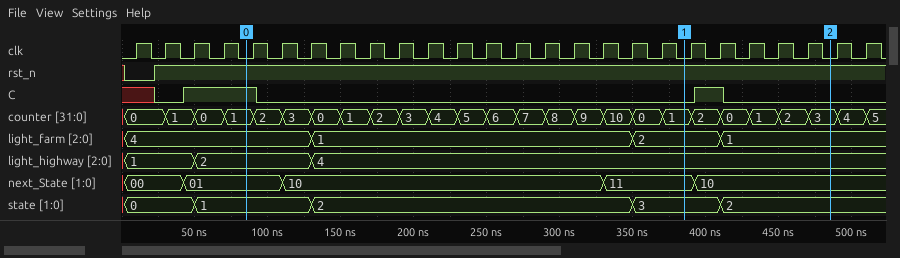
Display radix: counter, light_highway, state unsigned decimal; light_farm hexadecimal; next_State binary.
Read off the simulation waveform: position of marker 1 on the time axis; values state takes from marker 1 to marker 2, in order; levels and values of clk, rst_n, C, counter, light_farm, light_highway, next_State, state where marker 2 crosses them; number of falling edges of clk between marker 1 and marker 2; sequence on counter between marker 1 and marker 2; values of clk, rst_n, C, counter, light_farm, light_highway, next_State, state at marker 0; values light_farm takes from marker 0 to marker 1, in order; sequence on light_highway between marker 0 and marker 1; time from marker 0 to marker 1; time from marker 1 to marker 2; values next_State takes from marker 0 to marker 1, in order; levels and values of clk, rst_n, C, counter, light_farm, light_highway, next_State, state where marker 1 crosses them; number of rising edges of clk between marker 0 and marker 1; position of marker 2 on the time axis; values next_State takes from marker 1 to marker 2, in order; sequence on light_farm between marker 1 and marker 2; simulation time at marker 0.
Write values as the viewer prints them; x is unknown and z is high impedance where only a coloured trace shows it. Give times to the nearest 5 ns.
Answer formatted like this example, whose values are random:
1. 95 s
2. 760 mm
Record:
1. 385 ns
2. 3, 2
3. clk=0, rst_n=1, C=0, counter=3, light_farm=1, light_highway=4, next_State=10, state=2
4. 5
5. 1, 2, 0, 1, 2, 3
6. clk=0, rst_n=1, C=1, counter=1, light_farm=4, light_highway=2, next_State=01, state=1
7. 4, 1, 2
8. 2, 4
9. 300 ns
10. 100 ns
11. 01, 10, 11
12. clk=0, rst_n=1, C=0, counter=1, light_farm=2, light_highway=4, next_State=11, state=3
13. 15
14. 485 ns
15. 11, 10
16. 2, 1
17. 85 ns
